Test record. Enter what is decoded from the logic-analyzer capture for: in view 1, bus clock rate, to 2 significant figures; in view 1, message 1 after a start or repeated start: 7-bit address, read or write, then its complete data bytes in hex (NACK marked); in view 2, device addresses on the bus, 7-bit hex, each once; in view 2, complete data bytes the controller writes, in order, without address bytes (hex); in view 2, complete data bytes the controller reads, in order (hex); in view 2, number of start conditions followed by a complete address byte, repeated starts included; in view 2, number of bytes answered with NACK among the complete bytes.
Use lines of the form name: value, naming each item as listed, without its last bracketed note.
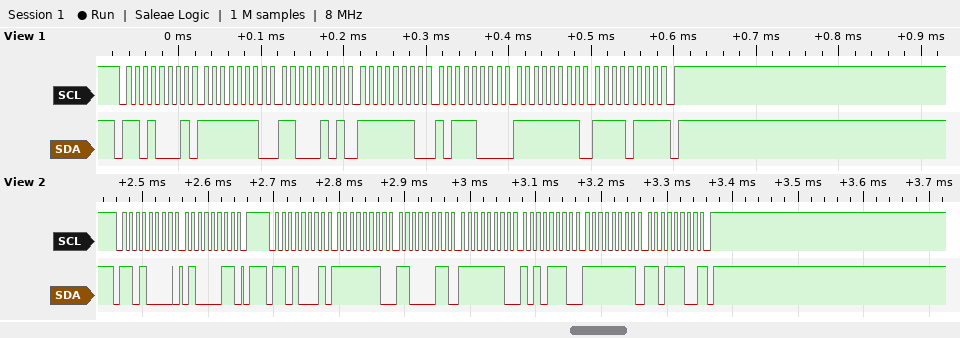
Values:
in view 1, bus clock rate, to 2 significant figures: 100 kHz
in view 1, message 1 after a start or repeated start: 7-bit address, read or write, then its complete data bytes in hex: 0x68 read: FE C5 FE B8 FF F7 NACK
in view 2, device addresses on the bus, 7-bit hex, each once: 0x68
in view 2, complete data bytes the controller writes, in order, without address bytes: 43
in view 2, complete data bytes the controller reads, in order: FE C3 FE AE FF DC
in view 2, number of start conditions followed by a complete address byte, repeated starts included: 2
in view 2, number of bytes answered with NACK among the complete bytes: 1
